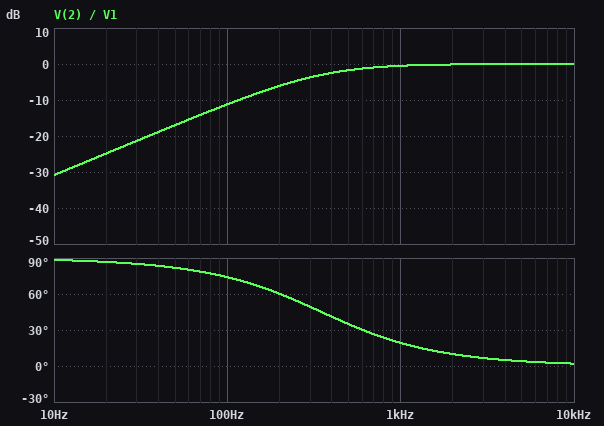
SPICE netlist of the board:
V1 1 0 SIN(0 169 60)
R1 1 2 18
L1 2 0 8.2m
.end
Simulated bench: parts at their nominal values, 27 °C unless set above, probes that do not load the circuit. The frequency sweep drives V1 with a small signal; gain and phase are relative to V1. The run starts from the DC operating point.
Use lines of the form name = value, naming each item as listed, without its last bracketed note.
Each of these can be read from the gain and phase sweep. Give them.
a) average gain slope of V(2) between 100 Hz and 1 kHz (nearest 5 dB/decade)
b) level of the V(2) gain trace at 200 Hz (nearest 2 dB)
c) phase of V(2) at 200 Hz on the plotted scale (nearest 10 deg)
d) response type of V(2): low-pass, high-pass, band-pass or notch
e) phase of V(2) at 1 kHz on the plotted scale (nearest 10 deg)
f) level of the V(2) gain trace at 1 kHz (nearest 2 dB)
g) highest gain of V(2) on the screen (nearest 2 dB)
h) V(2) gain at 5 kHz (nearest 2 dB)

average gain slope of V(2) between 100 Hz and 1 kHz = 10 dB/decade
level of the V(2) gain trace at 200 Hz = -6 dB
phase of V(2) at 200 Hz on the plotted scale = 60 deg
response type of V(2): low-pass, high-pass, band-pass or notch = high-pass
phase of V(2) at 1 kHz on the plotted scale = 20 deg
level of the V(2) gain trace at 1 kHz = 0 dB
highest gain of V(2) on the screen = 0 dB
V(2) gain at 5 kHz = 0 dB
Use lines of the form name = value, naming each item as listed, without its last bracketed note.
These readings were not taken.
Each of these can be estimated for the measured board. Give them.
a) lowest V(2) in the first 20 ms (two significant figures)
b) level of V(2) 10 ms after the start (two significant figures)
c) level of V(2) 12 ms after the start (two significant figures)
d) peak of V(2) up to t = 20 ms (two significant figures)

lowest V(2) in the first 20 ms = -29 V
level of V(2) 10 ms after the start = -26 V
level of V(2) 12 ms after the start = -10 V
peak of V(2) up to t = 20 ms = 29 V
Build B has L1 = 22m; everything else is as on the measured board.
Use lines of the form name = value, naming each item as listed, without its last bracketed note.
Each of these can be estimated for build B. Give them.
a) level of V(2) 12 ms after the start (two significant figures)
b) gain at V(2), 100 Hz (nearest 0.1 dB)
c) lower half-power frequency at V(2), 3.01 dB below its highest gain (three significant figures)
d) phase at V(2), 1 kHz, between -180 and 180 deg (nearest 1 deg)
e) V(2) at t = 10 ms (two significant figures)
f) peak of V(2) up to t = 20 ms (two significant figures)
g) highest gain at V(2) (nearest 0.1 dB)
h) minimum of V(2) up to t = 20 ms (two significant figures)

level of V(2) 12 ms after the start = -41 V
gain at V(2), 100 Hz = -4.3 dB
lower half-power frequency at V(2), 3.01 dB below its highest gain = 130 Hz
phase at V(2), 1 kHz, between -180 and 180 deg = 7 deg
V(2) at t = 10 ms = -69 V
peak of V(2) up to t = 20 ms = 71 V
highest gain at V(2) = 0 dB
minimum of V(2) up to t = 20 ms = -71 V
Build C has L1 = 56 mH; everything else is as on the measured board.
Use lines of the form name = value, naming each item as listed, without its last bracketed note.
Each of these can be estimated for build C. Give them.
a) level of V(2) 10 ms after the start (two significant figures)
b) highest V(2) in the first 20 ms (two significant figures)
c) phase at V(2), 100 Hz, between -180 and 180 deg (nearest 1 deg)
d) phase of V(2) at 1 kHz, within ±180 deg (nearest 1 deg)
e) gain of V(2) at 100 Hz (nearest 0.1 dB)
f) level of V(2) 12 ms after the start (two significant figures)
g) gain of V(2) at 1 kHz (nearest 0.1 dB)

level of V(2) 10 ms after the start = -130 V
highest V(2) in the first 20 ms = 130 V
phase at V(2), 100 Hz, between -180 and 180 deg = 27 deg
phase of V(2) at 1 kHz, within ±180 deg = 3 deg
gain of V(2) at 100 Hz = -1.0 dB
level of V(2) 12 ms after the start = -110 V
gain of V(2) at 1 kHz = 0 dB
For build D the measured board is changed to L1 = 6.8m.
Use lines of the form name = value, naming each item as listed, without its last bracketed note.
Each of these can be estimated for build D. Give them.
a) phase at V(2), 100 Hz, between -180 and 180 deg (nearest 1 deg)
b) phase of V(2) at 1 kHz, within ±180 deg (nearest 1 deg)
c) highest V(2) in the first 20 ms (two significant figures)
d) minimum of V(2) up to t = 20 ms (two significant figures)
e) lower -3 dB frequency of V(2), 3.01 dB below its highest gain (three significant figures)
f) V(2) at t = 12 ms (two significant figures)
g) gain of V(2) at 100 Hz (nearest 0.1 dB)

phase at V(2), 100 Hz, between -180 and 180 deg = 77 deg
phase of V(2) at 1 kHz, within ±180 deg = 23 deg
highest V(2) in the first 20 ms = 24 V
minimum of V(2) up to t = 20 ms = -24 V
lower -3 dB frequency of V(2), 3.01 dB below its highest gain = 421 Hz
V(2) at t = 12 ms = -7.7 V
gain of V(2) at 100 Hz = -12.7 dB
